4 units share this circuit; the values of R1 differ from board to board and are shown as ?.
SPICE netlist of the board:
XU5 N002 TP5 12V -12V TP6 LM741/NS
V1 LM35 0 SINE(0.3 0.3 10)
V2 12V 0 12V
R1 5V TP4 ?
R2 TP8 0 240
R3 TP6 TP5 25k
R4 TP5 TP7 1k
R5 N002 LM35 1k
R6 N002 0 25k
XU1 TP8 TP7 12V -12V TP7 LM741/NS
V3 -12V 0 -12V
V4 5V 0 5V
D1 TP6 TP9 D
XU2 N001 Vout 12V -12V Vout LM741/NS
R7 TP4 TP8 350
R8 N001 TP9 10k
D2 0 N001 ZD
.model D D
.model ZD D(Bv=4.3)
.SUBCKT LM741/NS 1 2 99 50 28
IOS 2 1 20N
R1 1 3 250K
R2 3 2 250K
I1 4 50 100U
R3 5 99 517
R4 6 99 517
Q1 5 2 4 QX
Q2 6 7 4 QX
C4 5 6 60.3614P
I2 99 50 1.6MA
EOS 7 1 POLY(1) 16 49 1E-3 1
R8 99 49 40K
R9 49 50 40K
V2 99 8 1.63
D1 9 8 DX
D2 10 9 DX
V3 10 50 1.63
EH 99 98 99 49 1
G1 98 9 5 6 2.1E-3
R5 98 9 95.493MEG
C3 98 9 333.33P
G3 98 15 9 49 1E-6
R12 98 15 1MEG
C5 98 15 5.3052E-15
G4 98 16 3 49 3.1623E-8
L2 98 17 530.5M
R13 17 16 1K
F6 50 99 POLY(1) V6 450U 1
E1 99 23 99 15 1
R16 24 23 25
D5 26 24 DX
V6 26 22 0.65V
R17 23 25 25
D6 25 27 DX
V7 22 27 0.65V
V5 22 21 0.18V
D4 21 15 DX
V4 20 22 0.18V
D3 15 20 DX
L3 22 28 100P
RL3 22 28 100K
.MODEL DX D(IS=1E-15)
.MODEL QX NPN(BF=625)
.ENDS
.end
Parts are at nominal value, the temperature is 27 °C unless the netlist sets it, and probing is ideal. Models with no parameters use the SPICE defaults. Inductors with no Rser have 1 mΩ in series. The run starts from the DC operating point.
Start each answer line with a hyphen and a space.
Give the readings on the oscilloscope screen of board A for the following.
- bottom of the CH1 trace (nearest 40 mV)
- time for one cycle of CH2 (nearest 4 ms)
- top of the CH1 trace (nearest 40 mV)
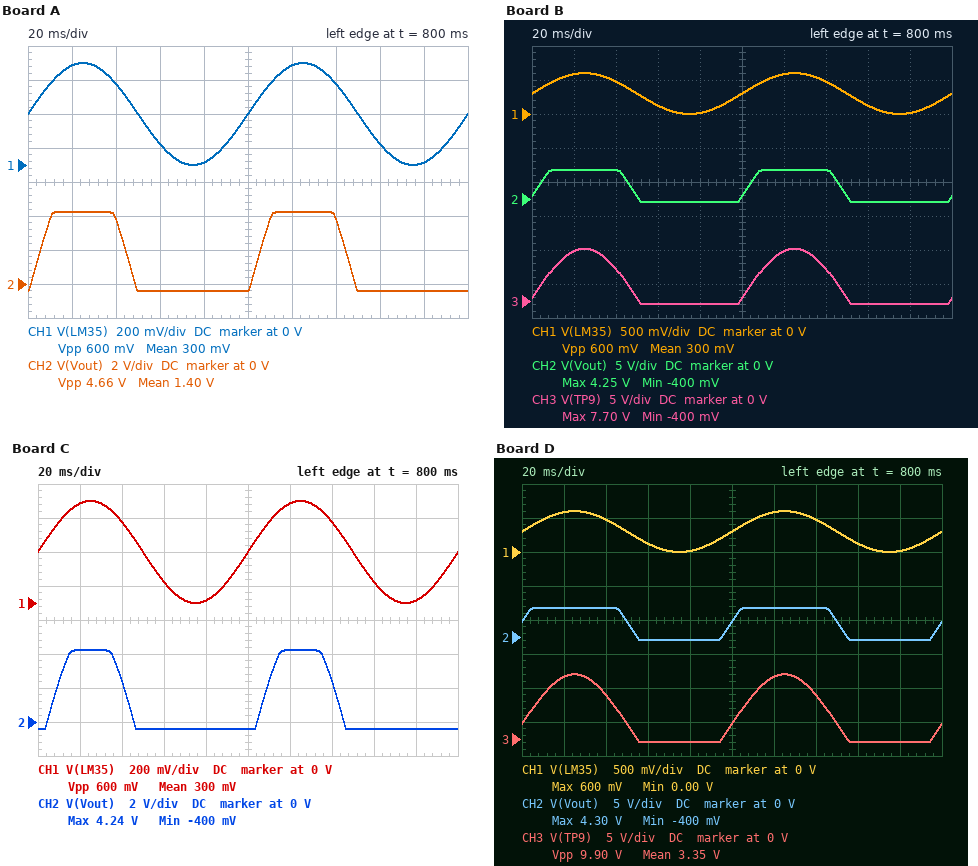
- 0 V
- 100 ms
- 600 mV
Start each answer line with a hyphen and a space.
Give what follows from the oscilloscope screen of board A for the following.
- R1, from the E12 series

- 3.3 kΩ
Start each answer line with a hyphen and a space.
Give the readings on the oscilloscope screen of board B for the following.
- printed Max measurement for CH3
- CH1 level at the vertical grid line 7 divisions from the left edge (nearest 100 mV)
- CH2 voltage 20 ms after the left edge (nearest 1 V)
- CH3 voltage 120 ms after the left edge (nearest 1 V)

- 7.70 V
- 500 mV
- 4 V
- 7 V
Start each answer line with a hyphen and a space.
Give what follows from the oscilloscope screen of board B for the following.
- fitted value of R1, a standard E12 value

- 3.9 kΩ
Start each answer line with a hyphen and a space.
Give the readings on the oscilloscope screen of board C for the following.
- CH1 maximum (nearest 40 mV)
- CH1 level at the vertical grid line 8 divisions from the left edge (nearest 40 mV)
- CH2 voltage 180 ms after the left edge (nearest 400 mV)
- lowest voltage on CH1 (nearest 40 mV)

- 600 mV
- 120 mV
- -400 mV
- 0 V
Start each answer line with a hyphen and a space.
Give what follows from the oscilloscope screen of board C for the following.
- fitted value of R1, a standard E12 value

- 2.7 kΩ
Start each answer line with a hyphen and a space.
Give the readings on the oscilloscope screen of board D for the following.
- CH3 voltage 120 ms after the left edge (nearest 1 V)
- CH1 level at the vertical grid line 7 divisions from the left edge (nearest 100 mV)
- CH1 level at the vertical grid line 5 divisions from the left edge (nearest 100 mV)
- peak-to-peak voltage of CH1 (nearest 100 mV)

- 9 V
- 500 mV
- 300 mV
- 600 mV
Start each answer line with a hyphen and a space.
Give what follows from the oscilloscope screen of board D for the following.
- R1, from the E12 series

- 5.6 kΩ
